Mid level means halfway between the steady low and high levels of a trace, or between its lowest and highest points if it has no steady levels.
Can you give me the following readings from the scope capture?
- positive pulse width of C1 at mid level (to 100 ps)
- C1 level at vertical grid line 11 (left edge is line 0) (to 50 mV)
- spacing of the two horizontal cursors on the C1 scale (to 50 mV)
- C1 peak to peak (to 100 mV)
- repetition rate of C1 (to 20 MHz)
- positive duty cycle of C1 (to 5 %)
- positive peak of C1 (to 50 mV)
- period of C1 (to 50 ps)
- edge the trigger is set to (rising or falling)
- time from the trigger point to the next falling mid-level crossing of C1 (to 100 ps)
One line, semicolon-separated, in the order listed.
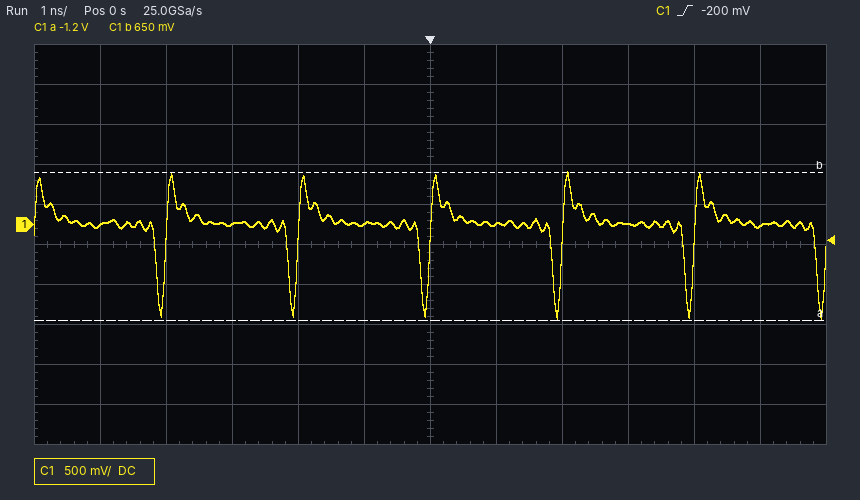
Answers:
1.8 ns; 0 mV; 1.85 V; 1.80 V; 500 MHz; 90 %; 650 mV; 2.00 ns; rising; 1.8 ns
